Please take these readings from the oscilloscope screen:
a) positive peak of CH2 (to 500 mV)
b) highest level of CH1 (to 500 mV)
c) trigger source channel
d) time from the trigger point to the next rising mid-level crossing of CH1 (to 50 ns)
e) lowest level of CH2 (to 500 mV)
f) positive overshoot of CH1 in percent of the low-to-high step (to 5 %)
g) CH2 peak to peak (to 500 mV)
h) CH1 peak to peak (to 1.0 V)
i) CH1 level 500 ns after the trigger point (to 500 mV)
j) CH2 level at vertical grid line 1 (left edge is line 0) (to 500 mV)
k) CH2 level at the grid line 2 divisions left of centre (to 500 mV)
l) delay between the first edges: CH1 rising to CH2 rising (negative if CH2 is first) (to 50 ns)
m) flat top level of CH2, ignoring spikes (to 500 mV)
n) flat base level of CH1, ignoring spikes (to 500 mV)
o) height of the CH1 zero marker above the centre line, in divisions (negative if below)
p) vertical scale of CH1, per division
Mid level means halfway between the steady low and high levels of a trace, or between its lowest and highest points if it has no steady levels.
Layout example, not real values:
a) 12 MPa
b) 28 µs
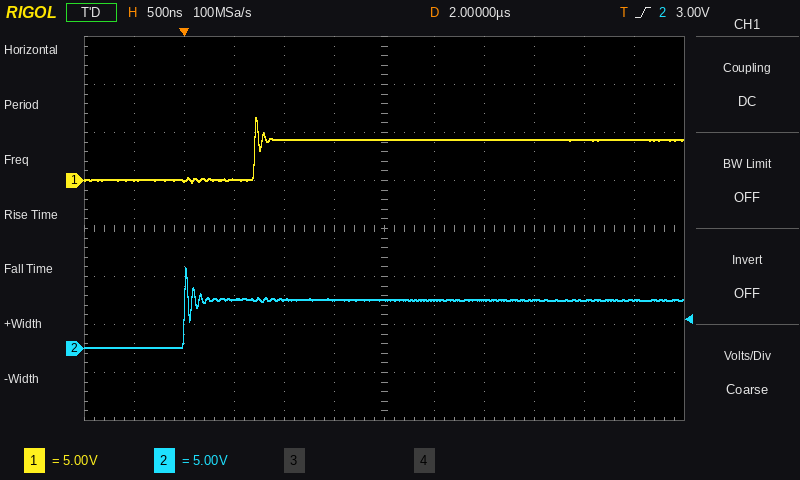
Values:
a) 8.5 V
b) 6.5 V
c) CH2
d) 700 ns
e) 0.0 V
f) 55 %
g) 8.5 V
h) 7.0 V
i) 0.0 V
j) 0.0 V
k) 5.0 V
l) -700 ns
m) 5.0 V
n) 0.0 V
o) +1.0 div
p) 5 V
